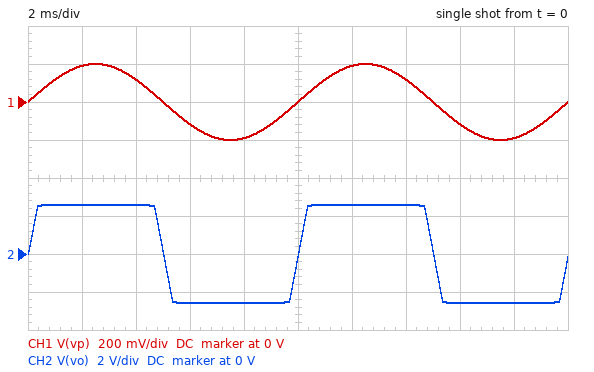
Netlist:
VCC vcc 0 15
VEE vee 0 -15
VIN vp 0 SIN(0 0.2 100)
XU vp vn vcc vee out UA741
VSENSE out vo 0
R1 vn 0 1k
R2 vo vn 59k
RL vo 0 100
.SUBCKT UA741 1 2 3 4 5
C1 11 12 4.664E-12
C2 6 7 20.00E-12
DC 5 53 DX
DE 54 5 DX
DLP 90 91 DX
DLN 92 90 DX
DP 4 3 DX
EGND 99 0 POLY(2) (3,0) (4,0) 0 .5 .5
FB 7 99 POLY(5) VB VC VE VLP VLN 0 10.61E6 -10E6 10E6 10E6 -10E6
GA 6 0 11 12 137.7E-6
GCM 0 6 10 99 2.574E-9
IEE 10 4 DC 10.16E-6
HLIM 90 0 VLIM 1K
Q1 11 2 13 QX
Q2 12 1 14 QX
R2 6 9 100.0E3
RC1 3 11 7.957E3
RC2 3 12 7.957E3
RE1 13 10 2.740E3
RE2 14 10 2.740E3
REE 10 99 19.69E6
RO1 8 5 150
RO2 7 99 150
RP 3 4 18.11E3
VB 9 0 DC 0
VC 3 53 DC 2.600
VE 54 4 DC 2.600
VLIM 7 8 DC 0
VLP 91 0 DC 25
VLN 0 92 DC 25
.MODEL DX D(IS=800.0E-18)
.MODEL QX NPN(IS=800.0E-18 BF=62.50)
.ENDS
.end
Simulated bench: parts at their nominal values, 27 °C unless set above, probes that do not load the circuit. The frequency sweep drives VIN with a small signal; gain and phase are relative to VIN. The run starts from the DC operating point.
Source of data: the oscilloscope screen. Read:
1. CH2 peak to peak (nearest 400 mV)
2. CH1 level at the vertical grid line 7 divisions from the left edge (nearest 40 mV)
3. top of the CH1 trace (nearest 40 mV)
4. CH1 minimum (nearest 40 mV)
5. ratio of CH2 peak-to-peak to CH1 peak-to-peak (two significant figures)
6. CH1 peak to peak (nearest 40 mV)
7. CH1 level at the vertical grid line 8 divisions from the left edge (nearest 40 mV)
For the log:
5.2 V
120 mV
200 mV
-200 mV
13
400 mV
-120 mV
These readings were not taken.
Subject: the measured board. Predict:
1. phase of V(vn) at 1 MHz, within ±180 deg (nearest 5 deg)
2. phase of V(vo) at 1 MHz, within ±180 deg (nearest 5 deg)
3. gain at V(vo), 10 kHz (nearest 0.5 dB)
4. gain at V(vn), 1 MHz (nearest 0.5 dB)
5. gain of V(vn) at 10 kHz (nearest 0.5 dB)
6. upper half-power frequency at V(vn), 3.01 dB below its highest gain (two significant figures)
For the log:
-105 deg
-115 deg
31.0 dB
-44.0 dB
-4.5 dB
7.3 kHz
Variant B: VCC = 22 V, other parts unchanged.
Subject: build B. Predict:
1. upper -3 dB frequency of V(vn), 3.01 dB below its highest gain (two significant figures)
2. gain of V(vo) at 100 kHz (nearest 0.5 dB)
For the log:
7.2 kHz
12.5 dB
